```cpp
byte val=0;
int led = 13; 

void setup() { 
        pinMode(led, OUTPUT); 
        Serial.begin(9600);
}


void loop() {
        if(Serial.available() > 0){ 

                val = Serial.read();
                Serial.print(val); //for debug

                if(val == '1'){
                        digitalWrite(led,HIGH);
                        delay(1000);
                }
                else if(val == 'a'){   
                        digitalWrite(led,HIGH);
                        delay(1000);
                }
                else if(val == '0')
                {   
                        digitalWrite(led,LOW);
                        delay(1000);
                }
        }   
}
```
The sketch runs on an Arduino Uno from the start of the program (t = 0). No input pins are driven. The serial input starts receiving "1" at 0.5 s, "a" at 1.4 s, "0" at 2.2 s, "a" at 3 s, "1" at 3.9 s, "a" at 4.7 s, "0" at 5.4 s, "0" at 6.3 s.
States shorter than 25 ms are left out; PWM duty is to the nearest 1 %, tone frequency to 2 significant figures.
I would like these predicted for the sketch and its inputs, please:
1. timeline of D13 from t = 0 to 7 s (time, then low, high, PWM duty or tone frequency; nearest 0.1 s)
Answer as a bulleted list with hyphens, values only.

- 0 s low; 0.5 s high; 2.5 s low; 3.5 s high; 6.5 s low
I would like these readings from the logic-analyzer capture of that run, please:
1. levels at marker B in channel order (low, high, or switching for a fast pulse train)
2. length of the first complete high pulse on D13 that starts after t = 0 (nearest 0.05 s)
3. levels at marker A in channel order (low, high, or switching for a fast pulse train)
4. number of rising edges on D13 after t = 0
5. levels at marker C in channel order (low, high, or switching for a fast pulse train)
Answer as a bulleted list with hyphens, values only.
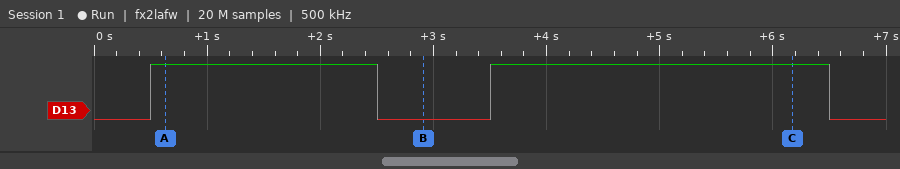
- D13 low
- 2.00 s
- D13 high
- 2
- D13 high
